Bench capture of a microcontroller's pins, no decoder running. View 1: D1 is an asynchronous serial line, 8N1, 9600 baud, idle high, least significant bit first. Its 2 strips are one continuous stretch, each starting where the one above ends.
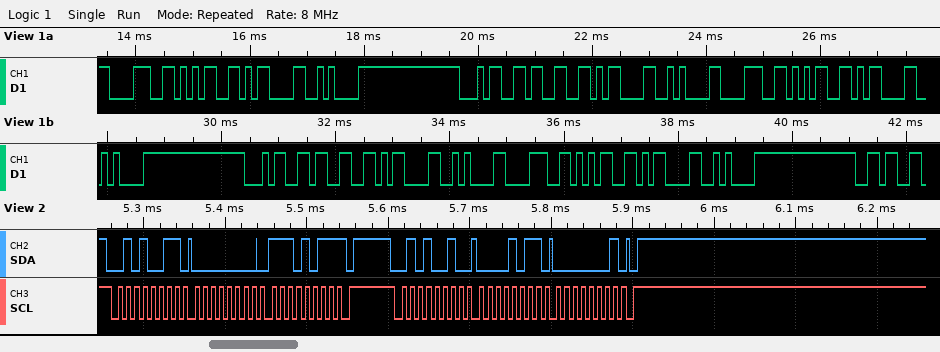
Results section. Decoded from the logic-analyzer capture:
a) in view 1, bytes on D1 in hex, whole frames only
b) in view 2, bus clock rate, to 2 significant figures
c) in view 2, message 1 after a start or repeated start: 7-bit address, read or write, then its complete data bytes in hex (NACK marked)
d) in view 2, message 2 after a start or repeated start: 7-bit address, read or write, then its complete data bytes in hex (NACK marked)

38 35 0D 0A 34 33 0D 0A 38 35 0D 0A 34 33 0D 0A 38 35 0D 0A 36
100 kHz
0x29 read: 00 EB NACK
0x29 write: 0B 01
